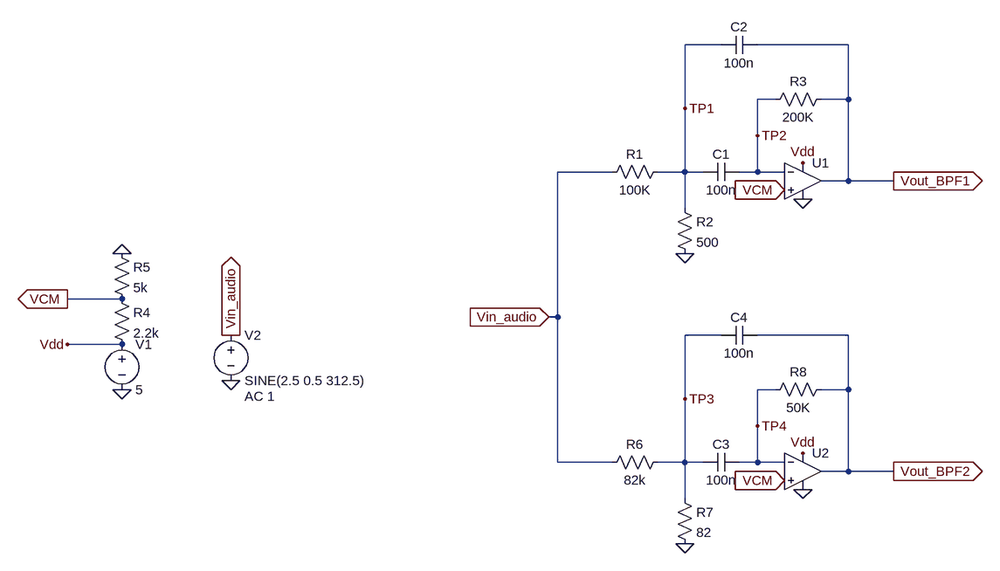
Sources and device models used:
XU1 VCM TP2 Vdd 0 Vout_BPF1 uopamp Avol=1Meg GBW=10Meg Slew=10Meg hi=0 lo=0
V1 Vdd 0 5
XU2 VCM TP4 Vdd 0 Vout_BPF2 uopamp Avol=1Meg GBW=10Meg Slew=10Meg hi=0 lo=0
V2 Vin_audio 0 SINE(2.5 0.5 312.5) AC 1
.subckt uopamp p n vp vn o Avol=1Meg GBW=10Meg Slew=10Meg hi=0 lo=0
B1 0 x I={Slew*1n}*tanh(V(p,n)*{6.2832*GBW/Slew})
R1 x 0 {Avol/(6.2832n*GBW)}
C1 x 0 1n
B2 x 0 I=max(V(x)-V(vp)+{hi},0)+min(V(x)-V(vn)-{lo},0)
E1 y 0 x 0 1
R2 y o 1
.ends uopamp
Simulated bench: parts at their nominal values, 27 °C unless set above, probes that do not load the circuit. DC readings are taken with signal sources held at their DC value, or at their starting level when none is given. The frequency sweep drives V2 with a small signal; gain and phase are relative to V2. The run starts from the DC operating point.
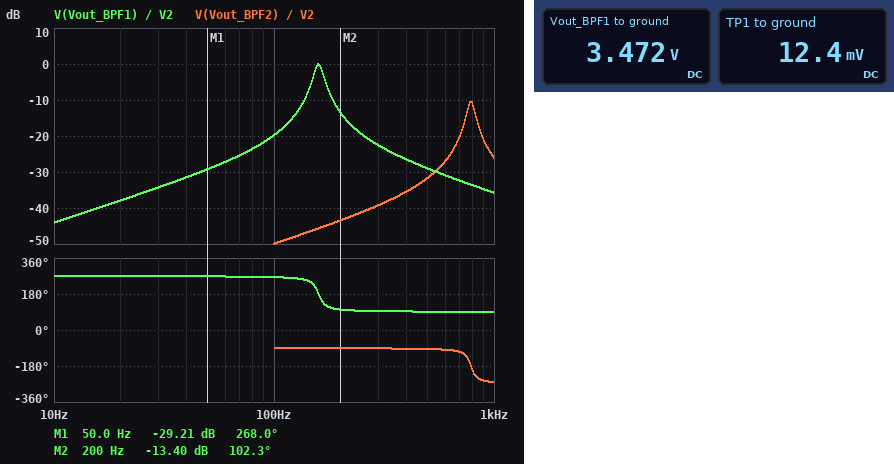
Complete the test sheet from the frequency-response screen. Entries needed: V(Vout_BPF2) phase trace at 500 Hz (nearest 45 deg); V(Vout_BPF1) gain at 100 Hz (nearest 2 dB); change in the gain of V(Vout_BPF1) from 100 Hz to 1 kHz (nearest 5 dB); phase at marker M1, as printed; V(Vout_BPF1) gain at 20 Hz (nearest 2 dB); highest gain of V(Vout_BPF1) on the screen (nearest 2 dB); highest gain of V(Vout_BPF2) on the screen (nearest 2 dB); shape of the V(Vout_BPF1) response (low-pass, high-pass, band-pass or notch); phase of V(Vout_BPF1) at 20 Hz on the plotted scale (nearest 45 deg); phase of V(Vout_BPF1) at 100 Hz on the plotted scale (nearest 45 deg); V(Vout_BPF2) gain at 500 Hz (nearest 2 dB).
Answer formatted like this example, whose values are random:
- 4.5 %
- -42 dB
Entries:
- -90 deg
- -20 dB
- -15 dB
- 268.0 deg
- -38 dB
- 0 dB
- -10 dB
- band-pass
- 270 deg
- 270 deg
- -32 dB
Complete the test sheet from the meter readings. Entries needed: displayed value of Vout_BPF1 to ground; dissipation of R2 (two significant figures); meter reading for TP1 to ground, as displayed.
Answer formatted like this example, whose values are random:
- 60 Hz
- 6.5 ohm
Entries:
- 3.472 V
- 310 nW
- 12.4 mV
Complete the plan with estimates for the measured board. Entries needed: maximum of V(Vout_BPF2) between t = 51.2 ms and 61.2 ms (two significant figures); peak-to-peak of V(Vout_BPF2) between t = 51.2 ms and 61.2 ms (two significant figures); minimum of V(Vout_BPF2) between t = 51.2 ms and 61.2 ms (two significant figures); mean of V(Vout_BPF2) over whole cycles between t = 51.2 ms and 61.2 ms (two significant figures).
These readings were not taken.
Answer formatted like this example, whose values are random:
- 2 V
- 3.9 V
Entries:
- 3.5 V
- 12 mV
- 3.5 V
- 3.5 V
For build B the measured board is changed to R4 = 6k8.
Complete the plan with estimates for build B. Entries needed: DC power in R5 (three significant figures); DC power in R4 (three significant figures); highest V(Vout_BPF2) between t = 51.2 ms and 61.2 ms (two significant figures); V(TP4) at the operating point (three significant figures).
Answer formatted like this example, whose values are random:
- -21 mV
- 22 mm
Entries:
- 898 µW
- 1.22 mW
- 2.1 V
- 2.12 V
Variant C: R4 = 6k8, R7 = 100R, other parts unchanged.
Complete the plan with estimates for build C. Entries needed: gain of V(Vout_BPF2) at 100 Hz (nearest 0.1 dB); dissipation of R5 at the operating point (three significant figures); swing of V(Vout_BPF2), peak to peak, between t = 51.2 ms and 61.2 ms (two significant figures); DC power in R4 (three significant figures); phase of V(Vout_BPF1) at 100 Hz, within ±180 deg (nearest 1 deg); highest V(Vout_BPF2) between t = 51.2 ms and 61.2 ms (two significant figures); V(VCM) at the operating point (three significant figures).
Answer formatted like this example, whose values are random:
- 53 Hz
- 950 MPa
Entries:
- -48.2 dB
- 898 µW
- 15 mV
- 1.22 mW
- -96 deg
- 2.1 V
- 2.12 V
